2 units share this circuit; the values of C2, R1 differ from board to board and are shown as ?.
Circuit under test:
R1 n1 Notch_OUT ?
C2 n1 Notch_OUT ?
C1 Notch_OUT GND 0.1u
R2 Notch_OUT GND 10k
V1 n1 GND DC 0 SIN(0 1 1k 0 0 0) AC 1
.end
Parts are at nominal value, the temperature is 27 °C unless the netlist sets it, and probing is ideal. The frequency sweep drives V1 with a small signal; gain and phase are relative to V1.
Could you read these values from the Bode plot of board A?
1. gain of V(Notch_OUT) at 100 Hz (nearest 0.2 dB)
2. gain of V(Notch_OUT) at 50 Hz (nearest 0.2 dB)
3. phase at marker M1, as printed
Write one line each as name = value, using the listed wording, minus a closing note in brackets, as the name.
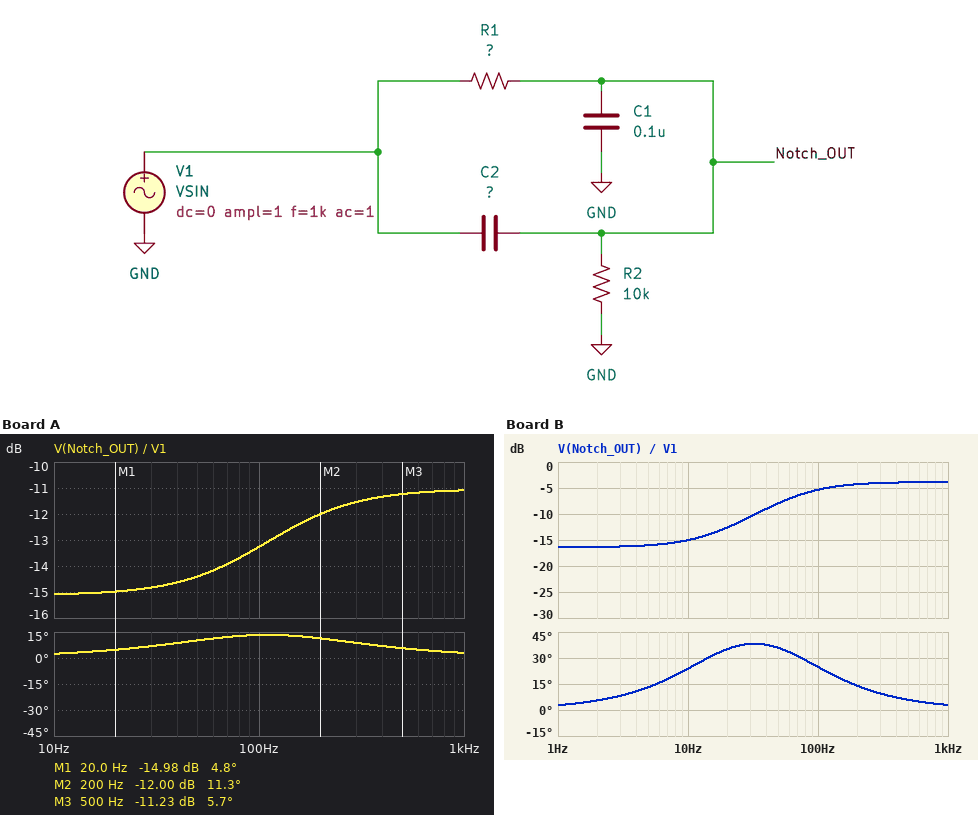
gain of V(Notch_OUT) at 100 Hz = -13.2 dB
gain of V(Notch_OUT) at 50 Hz = -14.4 dB
phase at marker M1, as printed = 4.8 deg
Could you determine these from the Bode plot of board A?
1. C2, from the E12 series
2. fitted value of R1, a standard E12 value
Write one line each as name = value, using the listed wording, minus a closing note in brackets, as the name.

C2, from the E12 series = 39 nF
fitted value of R1, a standard E12 value = 47 kΩ
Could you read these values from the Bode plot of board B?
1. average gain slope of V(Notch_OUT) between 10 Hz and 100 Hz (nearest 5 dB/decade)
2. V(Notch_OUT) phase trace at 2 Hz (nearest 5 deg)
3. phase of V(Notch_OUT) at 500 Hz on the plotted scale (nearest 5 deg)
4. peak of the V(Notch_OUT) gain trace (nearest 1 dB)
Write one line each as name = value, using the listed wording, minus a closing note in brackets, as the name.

average gain slope of V(Notch_OUT) between 10 Hz and 100 Hz = 10 dB/decade
V(Notch_OUT) phase trace at 2 Hz = 5 deg
phase of V(Notch_OUT) at 500 Hz on the plotted scale = 5 deg
peak of the V(Notch_OUT) gain trace = -4 dB
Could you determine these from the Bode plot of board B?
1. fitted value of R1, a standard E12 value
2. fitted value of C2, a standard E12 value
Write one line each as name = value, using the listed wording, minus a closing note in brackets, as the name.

fitted value of R1, a standard E12 value = 56 kΩ
fitted value of C2, a standard E12 value = 180 nF
